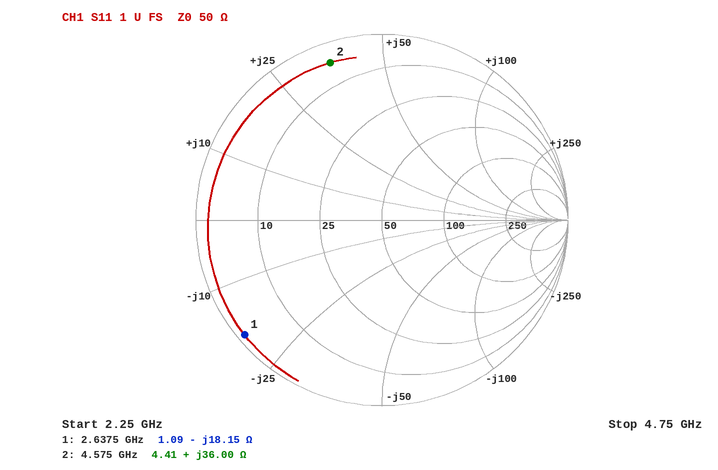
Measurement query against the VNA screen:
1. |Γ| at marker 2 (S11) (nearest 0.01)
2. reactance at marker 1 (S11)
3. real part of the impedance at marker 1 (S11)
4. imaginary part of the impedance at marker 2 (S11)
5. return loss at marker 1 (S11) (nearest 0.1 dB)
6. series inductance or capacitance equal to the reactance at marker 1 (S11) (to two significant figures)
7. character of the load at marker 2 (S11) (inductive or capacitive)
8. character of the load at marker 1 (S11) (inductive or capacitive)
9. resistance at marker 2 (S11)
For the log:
0.89
-18.15 Ω
1.09 Ω
+36.00 Ω
0.3 dB
3.3 pF
inductive
capacitive
4.41 Ω
